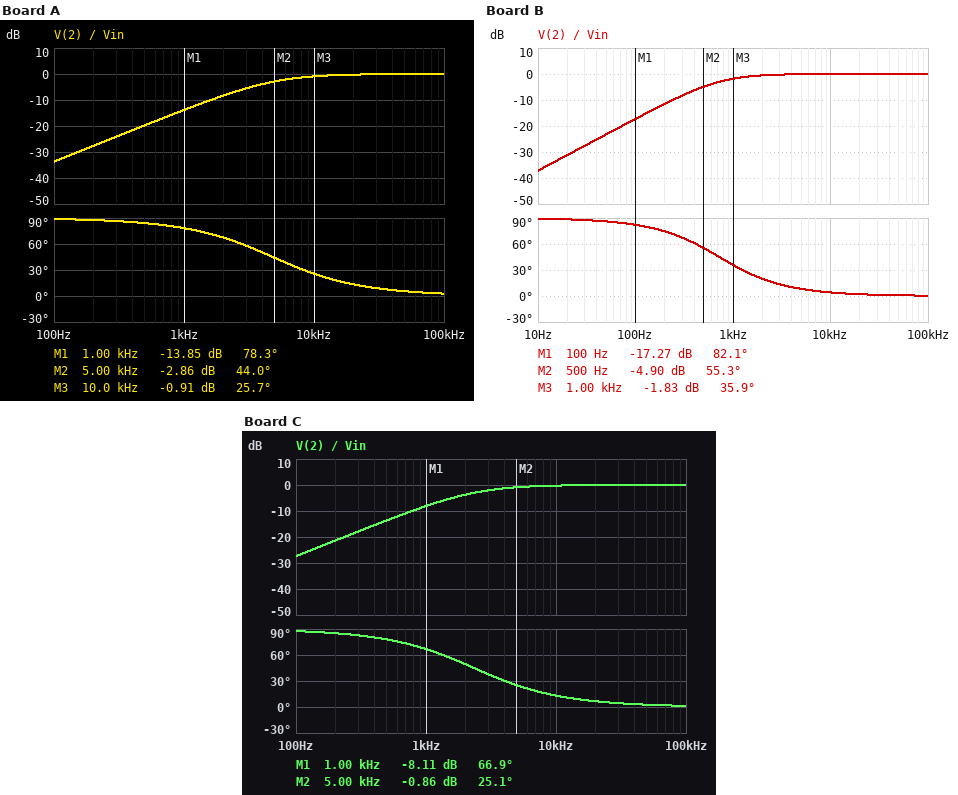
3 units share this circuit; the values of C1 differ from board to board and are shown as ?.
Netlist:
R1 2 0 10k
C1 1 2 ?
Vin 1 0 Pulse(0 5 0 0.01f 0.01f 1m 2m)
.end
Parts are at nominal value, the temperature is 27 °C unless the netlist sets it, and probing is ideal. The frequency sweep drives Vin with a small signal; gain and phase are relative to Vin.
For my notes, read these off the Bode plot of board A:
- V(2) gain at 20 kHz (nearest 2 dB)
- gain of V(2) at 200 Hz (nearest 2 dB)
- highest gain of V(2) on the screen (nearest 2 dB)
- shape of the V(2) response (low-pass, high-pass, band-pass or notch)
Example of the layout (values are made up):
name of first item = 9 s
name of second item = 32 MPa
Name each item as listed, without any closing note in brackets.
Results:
V(2) gain at 20 kHz = 0 dB
gain of V(2) at 200 Hz = -28 dB
highest gain of V(2) on the screen = 0 dB
shape of the V(2) response = high-pass
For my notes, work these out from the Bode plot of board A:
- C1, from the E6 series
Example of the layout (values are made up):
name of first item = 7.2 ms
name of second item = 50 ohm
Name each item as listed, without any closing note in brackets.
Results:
C1, from the E6 series = 3.3 nF
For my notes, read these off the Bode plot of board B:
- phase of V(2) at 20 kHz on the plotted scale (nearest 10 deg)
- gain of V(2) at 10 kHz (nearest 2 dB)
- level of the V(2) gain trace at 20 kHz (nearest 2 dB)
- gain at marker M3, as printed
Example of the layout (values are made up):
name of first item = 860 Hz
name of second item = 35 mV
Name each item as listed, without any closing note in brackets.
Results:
phase of V(2) at 20 kHz on the plotted scale = 0 deg
gain of V(2) at 10 kHz = 0 dB
level of the V(2) gain trace at 20 kHz = 0 dB
gain at marker M3, as printed = -1.83 dB
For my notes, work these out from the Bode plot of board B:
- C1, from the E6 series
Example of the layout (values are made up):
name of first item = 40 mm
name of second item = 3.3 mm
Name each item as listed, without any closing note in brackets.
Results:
C1, from the E6 series = 22 nF
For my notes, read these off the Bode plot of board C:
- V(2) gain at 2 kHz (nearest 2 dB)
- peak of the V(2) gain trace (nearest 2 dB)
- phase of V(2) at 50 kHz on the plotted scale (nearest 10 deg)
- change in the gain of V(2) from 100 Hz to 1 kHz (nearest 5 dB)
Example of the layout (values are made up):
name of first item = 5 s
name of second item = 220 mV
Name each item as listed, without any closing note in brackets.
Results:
V(2) gain at 2 kHz = -4 dB
peak of the V(2) gain trace = 0 dB
phase of V(2) at 50 kHz on the plotted scale = 0 deg
change in the gain of V(2) from 100 Hz to 1 kHz = 20 dB
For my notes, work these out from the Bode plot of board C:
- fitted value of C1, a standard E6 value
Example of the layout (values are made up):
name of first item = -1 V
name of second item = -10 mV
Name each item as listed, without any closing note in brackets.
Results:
fitted value of C1, a standard E6 value = 6.8 nF
